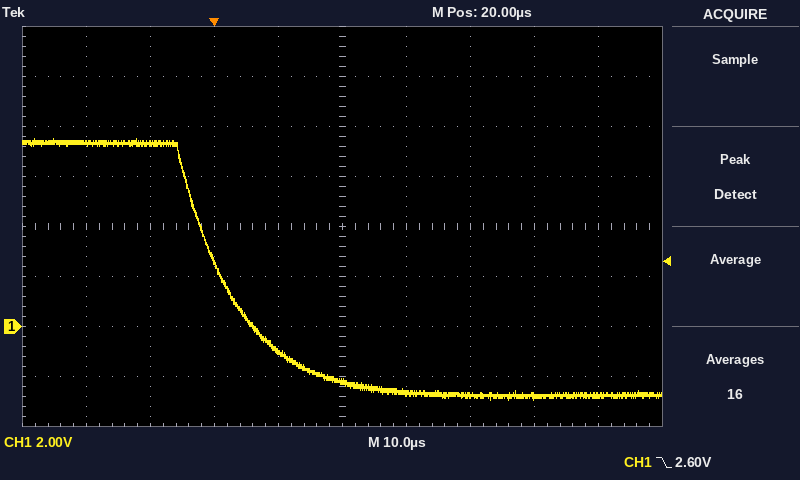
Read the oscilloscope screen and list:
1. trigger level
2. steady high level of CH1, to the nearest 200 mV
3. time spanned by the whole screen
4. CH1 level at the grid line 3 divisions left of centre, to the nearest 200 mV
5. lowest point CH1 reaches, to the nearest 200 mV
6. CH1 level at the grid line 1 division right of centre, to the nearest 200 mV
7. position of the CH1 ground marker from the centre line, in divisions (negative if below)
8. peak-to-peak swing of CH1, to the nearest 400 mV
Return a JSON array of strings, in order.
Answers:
["2.60 V", "7.4 V", "100 µs", "7.4 V", "-3.0 V", "-2.6 V", "-2.0 div", "10.4 V"]
